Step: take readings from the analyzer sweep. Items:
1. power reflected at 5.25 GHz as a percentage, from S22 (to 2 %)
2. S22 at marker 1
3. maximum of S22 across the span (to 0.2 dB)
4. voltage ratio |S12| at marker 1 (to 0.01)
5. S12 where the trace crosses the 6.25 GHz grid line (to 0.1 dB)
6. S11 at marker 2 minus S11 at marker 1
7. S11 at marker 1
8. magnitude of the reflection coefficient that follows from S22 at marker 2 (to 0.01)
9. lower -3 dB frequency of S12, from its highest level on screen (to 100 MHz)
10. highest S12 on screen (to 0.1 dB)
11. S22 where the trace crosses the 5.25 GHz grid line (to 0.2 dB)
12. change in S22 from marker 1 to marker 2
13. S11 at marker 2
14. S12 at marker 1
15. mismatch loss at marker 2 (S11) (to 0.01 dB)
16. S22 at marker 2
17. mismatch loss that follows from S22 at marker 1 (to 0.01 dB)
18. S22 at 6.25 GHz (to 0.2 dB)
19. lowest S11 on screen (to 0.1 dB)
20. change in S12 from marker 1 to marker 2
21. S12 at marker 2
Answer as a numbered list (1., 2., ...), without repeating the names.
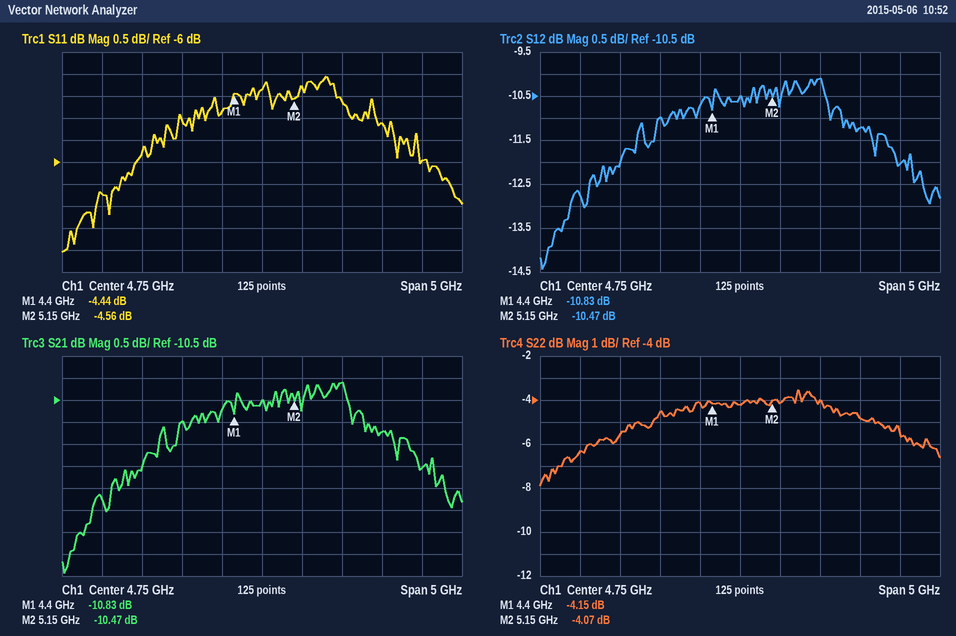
1. 38 %
2. -4.15 dB
3. -3.6 dB
4. 0.29
5. -11.2 dB
6. -0.12 dB
7. -4.44 dB
8. 0.63
9. 2.6 GHz
10. -10.1 dB
11. -4.2 dB
12. 0.08 dB
13. -4.56 dB
14. -10.83 dB
15. 1.87 dB
16. -4.07 dB
17. 2.11 dB
18. -4.8 dB
19. -8.0 dB
20. 0.36 dB
21. -10.47 dB
